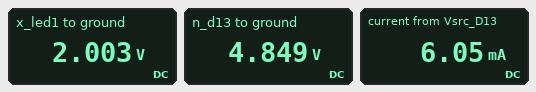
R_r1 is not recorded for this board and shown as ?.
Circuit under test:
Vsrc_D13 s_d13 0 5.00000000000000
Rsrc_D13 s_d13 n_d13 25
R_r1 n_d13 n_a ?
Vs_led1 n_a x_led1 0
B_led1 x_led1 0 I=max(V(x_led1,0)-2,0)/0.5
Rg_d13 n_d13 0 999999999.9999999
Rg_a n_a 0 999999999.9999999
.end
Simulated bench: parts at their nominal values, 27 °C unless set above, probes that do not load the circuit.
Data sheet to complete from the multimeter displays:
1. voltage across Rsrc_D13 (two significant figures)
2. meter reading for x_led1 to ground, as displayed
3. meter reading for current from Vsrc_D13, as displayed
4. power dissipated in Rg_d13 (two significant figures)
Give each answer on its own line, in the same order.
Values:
150 mV
2.003 V
6.05 mA
24 nW
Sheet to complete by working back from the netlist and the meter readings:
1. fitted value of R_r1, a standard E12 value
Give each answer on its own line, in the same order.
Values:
470 Ω
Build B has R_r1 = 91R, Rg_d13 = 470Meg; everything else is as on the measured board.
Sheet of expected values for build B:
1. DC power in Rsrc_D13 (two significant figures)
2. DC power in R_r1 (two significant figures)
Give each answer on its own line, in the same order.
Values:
17 mW
60 mW
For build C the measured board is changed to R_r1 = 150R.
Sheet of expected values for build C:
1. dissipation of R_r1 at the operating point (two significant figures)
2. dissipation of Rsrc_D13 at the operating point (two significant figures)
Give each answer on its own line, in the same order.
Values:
44 mW
7.3 mW
